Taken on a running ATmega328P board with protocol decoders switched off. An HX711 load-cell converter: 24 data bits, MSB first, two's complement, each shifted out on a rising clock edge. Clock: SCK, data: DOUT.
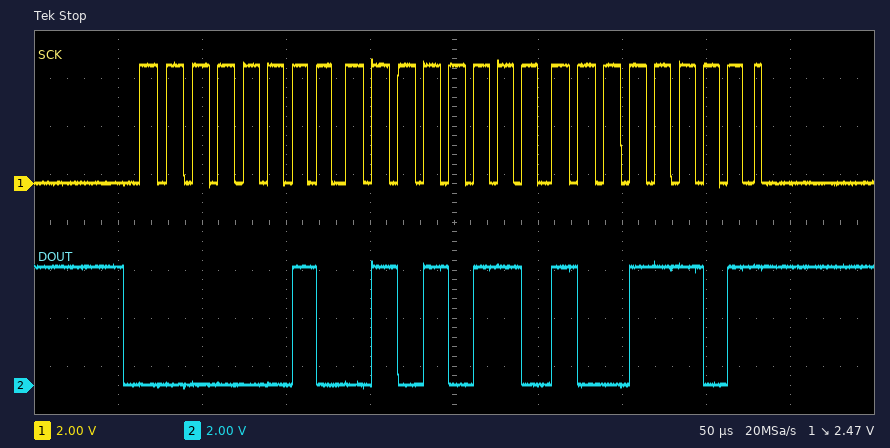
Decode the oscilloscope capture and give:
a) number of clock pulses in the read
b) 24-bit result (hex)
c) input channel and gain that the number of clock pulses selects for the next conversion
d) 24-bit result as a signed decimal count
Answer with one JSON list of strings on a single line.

["25", "0x02569D", "channel A, gain 128", "153245"]
